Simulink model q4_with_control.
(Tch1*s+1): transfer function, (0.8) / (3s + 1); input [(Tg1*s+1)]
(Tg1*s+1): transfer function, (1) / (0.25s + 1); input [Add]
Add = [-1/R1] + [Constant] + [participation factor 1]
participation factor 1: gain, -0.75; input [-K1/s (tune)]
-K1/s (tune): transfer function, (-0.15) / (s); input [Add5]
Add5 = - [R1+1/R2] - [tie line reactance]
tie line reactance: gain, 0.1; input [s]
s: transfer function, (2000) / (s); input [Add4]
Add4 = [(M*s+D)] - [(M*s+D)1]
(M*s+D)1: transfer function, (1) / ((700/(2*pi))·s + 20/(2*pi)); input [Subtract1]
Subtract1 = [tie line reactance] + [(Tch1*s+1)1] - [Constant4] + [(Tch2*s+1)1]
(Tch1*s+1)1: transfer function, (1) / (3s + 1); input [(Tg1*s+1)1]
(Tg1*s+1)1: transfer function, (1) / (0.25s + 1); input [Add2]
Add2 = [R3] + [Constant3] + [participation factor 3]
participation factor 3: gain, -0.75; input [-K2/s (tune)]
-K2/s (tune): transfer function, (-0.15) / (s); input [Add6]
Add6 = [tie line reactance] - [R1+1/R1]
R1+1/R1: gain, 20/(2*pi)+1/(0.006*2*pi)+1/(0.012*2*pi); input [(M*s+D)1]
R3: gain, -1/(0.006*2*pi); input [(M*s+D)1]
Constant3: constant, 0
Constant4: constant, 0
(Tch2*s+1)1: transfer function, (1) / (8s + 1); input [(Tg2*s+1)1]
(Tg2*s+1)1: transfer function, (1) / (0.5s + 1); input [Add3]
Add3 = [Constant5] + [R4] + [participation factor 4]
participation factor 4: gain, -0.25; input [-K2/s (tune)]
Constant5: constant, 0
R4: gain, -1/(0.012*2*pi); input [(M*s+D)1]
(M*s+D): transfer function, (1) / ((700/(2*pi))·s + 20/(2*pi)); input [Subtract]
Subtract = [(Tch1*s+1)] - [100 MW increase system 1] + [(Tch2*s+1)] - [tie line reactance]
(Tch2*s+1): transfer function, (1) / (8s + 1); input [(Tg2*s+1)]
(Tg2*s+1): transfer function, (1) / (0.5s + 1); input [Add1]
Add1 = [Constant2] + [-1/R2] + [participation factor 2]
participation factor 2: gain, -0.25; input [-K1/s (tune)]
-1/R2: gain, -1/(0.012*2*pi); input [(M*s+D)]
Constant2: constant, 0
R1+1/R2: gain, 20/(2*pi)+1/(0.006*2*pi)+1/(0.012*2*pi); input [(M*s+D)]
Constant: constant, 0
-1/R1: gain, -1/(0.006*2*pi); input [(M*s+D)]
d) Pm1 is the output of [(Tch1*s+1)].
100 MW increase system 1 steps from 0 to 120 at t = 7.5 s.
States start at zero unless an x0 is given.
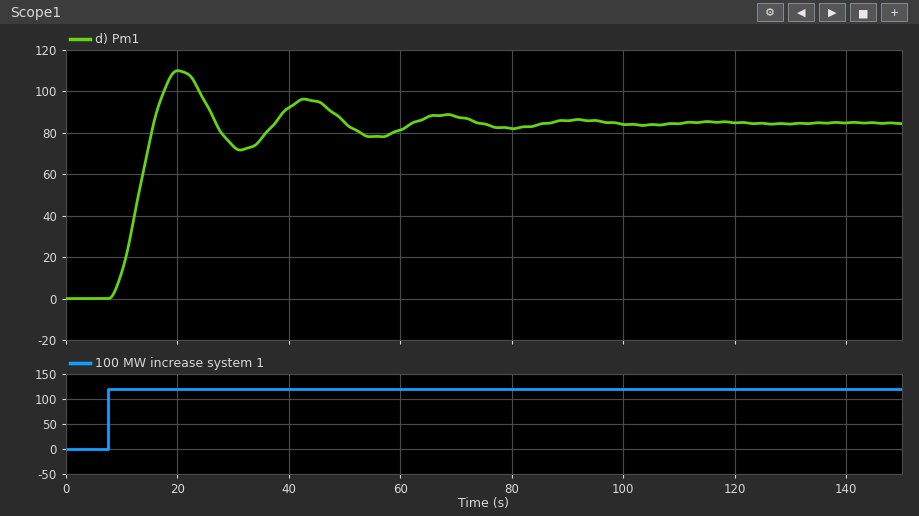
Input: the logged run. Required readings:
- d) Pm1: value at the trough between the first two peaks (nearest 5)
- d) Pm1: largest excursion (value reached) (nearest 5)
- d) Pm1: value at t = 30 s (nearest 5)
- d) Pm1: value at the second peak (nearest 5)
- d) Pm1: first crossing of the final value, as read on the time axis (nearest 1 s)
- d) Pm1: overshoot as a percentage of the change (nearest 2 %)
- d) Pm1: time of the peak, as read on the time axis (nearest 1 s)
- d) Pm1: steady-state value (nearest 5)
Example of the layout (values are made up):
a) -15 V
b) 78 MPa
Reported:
a) 70
b) 110
c) 75
d) 95
e) 16 s
f) 30 %
g) 20 s
h) 85
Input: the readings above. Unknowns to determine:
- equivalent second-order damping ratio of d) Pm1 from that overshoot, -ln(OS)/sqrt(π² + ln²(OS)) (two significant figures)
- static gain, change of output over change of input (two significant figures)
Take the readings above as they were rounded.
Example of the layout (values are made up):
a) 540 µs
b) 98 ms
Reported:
a) 0.36
b) 0.71
